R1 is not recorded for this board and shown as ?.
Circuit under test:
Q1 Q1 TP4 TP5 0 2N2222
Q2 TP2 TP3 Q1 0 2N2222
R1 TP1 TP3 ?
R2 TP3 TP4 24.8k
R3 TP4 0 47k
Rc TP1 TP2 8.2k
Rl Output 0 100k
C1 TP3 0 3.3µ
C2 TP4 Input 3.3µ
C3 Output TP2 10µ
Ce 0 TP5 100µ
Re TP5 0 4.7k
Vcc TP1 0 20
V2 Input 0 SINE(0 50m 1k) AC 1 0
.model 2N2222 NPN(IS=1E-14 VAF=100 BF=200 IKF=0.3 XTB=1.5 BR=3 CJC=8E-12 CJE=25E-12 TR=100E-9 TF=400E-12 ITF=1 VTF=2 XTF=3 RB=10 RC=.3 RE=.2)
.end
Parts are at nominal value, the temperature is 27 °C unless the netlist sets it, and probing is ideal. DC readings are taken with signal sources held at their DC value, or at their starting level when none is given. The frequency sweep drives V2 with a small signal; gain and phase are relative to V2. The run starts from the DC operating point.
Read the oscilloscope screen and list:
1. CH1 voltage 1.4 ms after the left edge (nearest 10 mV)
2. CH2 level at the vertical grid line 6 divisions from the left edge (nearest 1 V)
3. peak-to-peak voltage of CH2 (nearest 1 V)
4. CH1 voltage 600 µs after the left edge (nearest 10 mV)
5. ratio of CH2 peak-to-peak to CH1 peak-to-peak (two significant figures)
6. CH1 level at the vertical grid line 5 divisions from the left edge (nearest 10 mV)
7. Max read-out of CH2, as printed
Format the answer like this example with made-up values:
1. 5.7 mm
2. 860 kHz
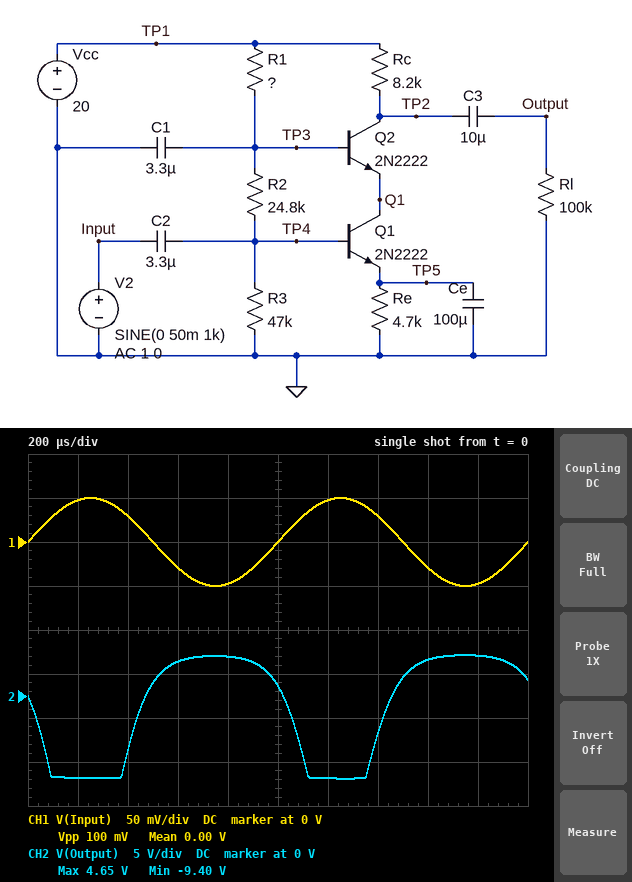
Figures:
1. 30 mV
2. -9 V
3. 14 V
4. -30 mV
5. 140
6. 0 V
7. 4.65 V
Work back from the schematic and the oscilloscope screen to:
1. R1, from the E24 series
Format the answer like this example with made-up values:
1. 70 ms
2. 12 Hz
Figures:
1. 160 kΩ
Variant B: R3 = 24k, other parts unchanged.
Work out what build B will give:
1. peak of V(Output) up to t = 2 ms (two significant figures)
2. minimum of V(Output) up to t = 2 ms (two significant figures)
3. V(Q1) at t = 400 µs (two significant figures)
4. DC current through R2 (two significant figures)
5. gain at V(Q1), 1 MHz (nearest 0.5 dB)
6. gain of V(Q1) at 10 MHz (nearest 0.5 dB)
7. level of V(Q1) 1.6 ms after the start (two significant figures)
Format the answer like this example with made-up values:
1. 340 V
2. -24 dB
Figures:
1. 2.3 V
2. -13 V
3. 3.9 V
4. 95 µA
5. 0 dB
6. 0.5 dB
7. 4.0 V
